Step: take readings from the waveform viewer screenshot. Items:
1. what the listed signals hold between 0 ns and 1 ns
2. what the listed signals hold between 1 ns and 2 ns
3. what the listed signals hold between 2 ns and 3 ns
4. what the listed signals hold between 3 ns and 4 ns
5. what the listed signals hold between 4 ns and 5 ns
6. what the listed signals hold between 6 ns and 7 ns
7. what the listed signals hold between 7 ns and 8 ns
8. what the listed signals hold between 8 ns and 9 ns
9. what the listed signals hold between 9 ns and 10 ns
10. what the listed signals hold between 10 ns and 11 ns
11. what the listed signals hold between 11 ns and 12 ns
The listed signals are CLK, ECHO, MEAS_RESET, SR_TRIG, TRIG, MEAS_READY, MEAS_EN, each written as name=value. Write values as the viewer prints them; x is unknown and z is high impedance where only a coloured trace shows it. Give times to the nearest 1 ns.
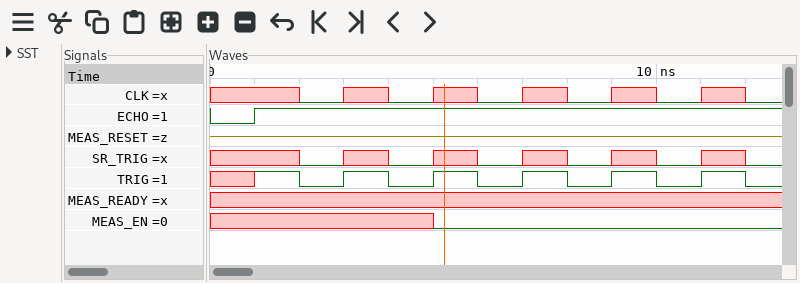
CLK=x, ECHO=0, MEAS_RESET=z, SR_TRIG=x, TRIG=x, MEAS_READY=x, MEAS_EN=x
CLK=x, ECHO=1, MEAS_RESET=z, SR_TRIG=x, TRIG=1, MEAS_READY=x, MEAS_EN=x
CLK=0, ECHO=1, MEAS_RESET=z, SR_TRIG=0, TRIG=0, MEAS_READY=x, MEAS_EN=x
CLK=x, ECHO=1, MEAS_RESET=z, SR_TRIG=x, TRIG=1, MEAS_READY=x, MEAS_EN=x
CLK=0, ECHO=1, MEAS_RESET=z, SR_TRIG=0, TRIG=0, MEAS_READY=x, MEAS_EN=x
CLK=0, ECHO=1, MEAS_RESET=z, SR_TRIG=0, TRIG=0, MEAS_READY=x, MEAS_EN=0
CLK=x, ECHO=1, MEAS_RESET=z, SR_TRIG=x, TRIG=1, MEAS_READY=x, MEAS_EN=0
CLK=0, ECHO=1, MEAS_RESET=z, SR_TRIG=0, TRIG=0, MEAS_READY=x, MEAS_EN=0
CLK=x, ECHO=1, MEAS_RESET=z, SR_TRIG=x, TRIG=1, MEAS_READY=x, MEAS_EN=0
CLK=0, ECHO=1, MEAS_RESET=z, SR_TRIG=0, TRIG=0, MEAS_READY=x, MEAS_EN=0
CLK=x, ECHO=1, MEAS_RESET=z, SR_TRIG=x, TRIG=1, MEAS_READY=x, MEAS_EN=0
